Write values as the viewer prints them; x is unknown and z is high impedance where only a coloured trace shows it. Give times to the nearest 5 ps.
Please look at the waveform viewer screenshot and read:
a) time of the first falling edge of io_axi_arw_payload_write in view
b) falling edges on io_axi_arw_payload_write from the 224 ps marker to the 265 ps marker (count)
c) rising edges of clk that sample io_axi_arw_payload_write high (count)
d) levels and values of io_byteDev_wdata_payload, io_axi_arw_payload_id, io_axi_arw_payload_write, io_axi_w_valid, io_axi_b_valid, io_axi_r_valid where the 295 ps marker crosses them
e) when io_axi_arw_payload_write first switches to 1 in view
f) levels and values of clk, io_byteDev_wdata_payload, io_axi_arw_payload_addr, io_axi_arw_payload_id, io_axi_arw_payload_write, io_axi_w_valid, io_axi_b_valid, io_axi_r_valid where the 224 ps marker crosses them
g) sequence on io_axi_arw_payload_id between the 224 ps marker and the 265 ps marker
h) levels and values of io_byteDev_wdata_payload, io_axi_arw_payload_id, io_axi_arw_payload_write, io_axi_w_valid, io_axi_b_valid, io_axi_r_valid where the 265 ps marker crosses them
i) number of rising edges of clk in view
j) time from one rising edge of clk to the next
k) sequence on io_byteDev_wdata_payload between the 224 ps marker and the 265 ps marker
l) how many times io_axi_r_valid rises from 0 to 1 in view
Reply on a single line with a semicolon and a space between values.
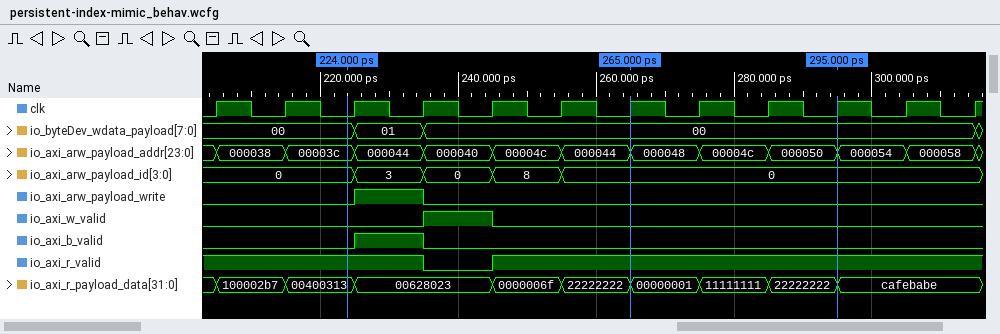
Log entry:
235 ps; 1; 1; io_byteDev_wdata_payload=00, io_axi_arw_payload_id=0, io_axi_arw_payload_write=0, io_axi_w_valid=0, io_axi_b_valid=0, io_axi_r_valid=1; 225 ps; clk=0, io_byteDev_wdata_payload=00, io_axi_arw_payload_addr=00003c, io_axi_arw_payload_id=0, io_axi_arw_payload_write=0, io_axi_w_valid=0, io_axi_b_valid=0, io_axi_r_valid=1; 0, 3, 0, 8, 0; io_byteDev_wdata_payload=00, io_axi_arw_payload_id=0, io_axi_arw_payload_write=0, io_axi_w_valid=0, io_axi_b_valid=0, io_axi_r_valid=1; 12; 10 ps; 00, 01, 00; 1
